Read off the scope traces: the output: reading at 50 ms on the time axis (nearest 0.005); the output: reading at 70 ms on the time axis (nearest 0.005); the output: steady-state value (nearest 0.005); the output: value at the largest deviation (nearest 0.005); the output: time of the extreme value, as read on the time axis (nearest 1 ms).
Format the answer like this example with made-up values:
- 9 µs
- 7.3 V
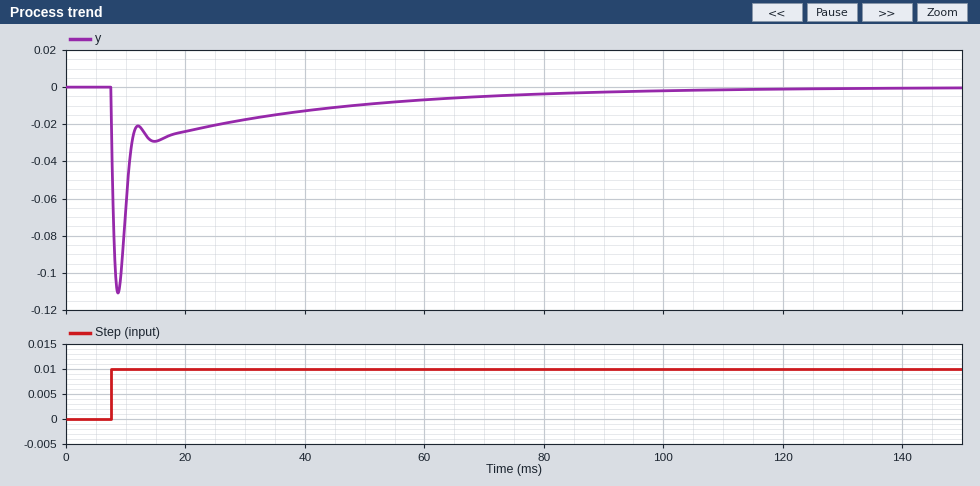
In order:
- -0.010
- -0.005
- 0.000
- -0.110
- 9 ms
